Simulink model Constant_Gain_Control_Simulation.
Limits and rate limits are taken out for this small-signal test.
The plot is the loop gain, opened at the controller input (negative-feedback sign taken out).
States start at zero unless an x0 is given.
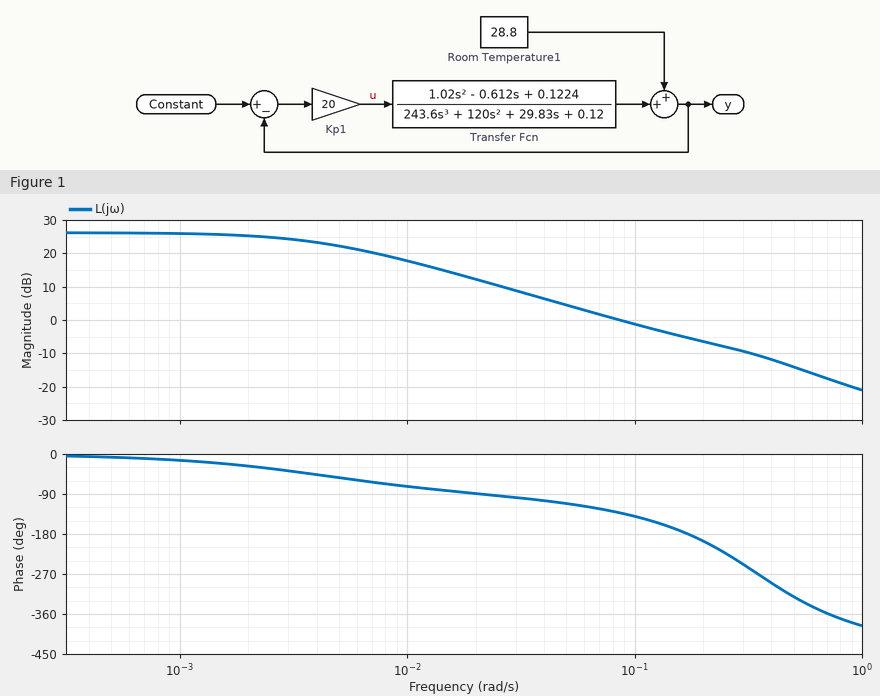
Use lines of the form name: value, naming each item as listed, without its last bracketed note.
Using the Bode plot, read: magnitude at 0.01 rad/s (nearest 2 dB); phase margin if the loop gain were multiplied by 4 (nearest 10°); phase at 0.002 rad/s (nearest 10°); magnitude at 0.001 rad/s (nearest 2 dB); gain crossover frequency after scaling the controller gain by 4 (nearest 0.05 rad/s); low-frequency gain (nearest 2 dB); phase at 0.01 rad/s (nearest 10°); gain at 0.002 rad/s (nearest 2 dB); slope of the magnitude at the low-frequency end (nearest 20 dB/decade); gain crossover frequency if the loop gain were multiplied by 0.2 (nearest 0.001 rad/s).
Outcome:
magnitude at 0.01 rad/s: 18 dB
phase margin if the loop gain were multiplied by 4: -110°
phase at 0.002 rad/s: -30°
magnitude at 0.001 rad/s: 26 dB
gain crossover frequency after scaling the controller gain by 4: 0.40 rad/s
low-frequency gain: 26 dB
phase at 0.01 rad/s: -70°
gain at 0.002 rad/s: 26 dB
slope of the magnitude at the low-frequency end: 0 dB/decade
gain crossover frequency if the loop gain were multiplied by 0.2: 0.016 rad/s
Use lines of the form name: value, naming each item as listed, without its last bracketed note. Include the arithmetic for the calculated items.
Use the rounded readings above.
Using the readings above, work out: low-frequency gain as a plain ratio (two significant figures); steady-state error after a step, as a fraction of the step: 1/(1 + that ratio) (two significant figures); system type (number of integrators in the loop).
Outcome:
low-frequency gain as a plain ratio: 10^(26 / 20) = 20
steady-state error after a step, as a fraction of the step: 1/(1 + that ratio): 1 / (1 + 20) = 0.048
system type: 0
